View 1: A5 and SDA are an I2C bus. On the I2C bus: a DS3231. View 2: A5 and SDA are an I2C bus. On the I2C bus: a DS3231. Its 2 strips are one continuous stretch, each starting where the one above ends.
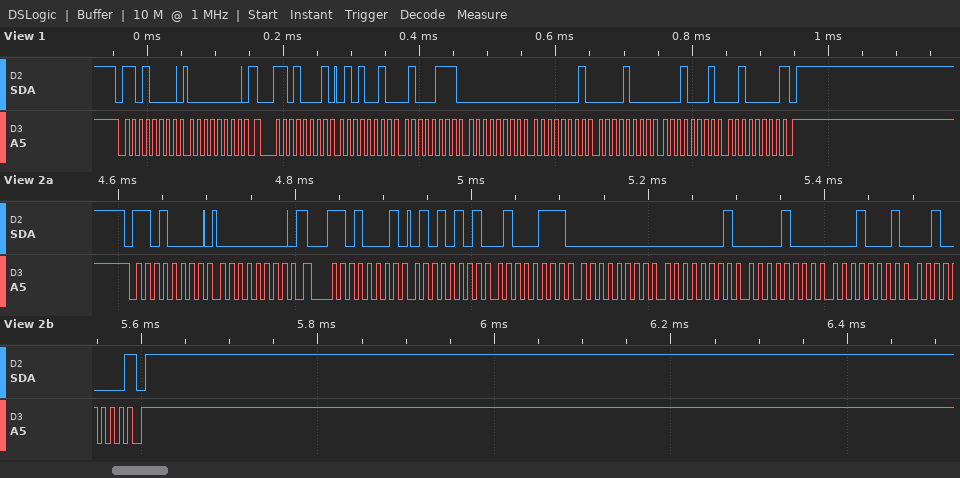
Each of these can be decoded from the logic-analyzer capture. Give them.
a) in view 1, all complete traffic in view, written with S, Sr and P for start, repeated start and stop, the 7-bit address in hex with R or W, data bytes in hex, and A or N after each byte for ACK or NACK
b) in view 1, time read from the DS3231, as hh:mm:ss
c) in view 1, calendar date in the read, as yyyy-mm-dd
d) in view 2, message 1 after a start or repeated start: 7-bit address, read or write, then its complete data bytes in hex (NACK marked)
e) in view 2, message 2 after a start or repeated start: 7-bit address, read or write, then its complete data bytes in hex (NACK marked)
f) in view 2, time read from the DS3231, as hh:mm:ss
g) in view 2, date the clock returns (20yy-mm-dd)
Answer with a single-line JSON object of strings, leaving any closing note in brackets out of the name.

{"in view 1, all complete traffic in view, written with S, Sr and P for start, repeated start and stop, the 7-bit address in hex with R or W, data bytes in hex, and A or N after each byte for ACK or NACK": "S 68W A 00 A Sr 68R A 52 A 47 A 00 A 01 A 08 A 11 A 20 N P", "in view 1, time read from the DS3231, as hh:mm:ss": "00:47:52", "in view 1, calendar date in the read, as yyyy-mm-dd": "2020-11-08", "in view 2, message 1 after a start or repeated start: 7-bit address, read or write, then its complete data bytes in hex": "0x68 write: 00", "in view 2, message 2 after a start or repeated start: 7-bit address, read or write, then its complete data bytes in hex": "0x68 read: 55 47 00 01 08 11 20 NACK", "in view 2, time read from the DS3231, as hh:mm:ss": "00:47:55", "in view 2, date the clock returns": "2020-11-08"}
